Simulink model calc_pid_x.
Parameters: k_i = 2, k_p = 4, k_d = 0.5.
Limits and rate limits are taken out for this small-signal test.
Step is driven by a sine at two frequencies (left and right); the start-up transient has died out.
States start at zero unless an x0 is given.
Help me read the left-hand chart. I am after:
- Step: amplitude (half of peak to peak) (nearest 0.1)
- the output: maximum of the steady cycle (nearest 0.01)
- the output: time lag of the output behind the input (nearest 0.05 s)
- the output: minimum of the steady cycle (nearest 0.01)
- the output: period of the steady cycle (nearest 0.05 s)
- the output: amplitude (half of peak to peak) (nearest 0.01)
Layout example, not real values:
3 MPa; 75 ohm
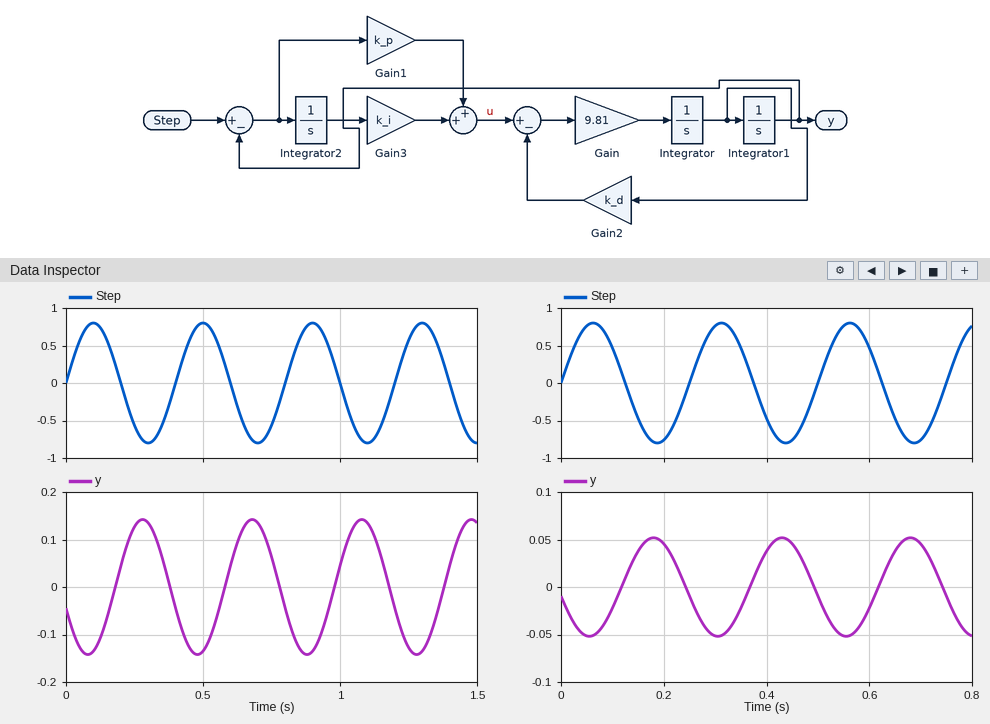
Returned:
0.8; 0.14; 0.20 s; -0.14; 0.40 s; 0.14
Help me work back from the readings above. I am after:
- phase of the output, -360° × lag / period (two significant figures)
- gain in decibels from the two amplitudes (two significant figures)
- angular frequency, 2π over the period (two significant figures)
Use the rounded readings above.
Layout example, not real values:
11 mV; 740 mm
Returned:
-180°; -15 dB; 16 rad/s
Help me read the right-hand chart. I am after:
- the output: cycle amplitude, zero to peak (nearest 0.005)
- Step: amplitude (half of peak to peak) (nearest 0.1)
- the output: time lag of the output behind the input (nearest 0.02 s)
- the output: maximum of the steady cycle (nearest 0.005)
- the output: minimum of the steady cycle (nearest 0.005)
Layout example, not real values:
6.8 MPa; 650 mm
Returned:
0.050; 0.8; 0.12 s; 0.050; -0.050
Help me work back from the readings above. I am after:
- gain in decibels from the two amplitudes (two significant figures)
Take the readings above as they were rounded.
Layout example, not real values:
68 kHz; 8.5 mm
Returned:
-24 dB
